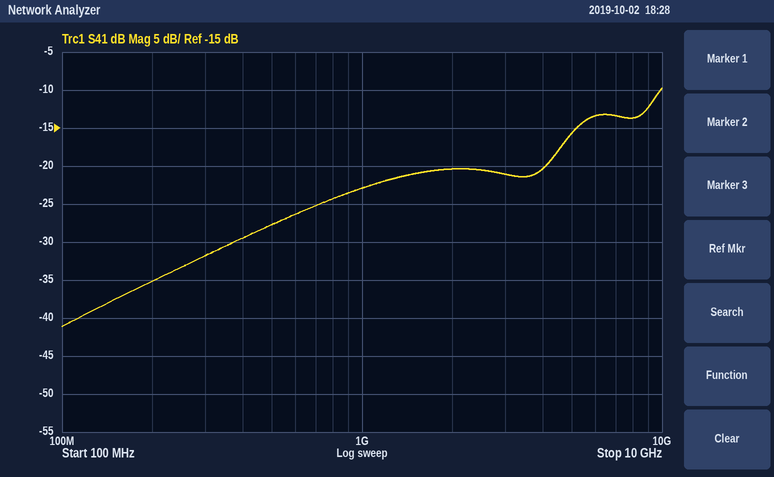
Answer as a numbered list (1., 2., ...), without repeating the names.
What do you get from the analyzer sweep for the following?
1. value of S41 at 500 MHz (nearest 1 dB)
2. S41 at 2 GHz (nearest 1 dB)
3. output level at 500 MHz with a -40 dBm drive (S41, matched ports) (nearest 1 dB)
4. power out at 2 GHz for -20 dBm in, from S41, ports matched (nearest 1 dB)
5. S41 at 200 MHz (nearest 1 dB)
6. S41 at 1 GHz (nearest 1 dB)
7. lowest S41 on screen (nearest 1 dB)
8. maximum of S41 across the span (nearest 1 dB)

1. -28 dB
2. -20 dB
3. -68 dBm
4. -40 dBm
5. -35 dB
6. -23 dB
7. -41 dB
8. -10 dB
